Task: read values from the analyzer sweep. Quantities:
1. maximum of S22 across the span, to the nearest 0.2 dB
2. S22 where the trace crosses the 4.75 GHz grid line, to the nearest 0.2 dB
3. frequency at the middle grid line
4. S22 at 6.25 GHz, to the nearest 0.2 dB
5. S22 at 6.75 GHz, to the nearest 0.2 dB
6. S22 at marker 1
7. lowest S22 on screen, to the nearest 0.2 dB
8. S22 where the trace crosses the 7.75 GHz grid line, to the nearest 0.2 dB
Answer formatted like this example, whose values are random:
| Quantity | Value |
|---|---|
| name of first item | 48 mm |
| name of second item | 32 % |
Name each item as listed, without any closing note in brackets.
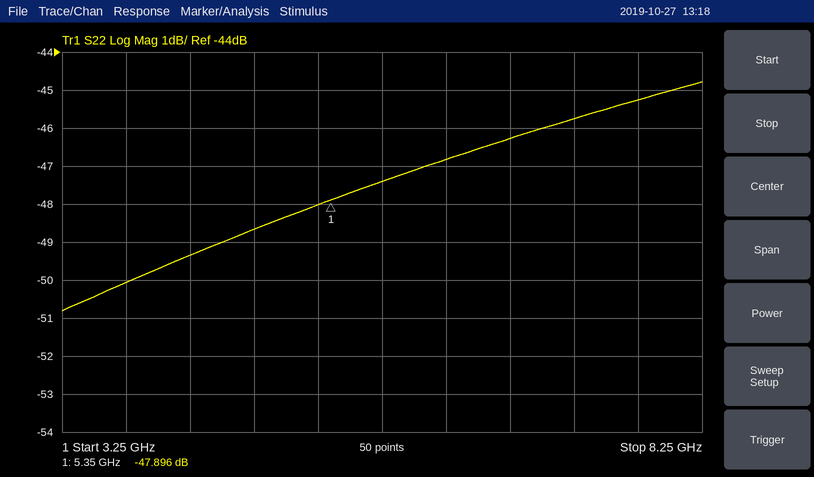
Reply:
| Quantity | Value |
|---|---|
| maximum of S22 across the span, to the nearest 0.2 dB | -44.8 dB |
| S22 where the trace crosses the 4.75 GHz grid line, to the nearest 0.2 dB | -48.6 dB |
| frequency at the middle grid line | 5.75 GHz |
| S22 at 6.25 GHz, to the nearest 0.2 dB | -46.8 dB |
| S22 at 6.75 GHz, to the nearest 0.2 dB | -46.2 dB |
| S22 at marker 1 | -47.896 dB |
| lowest S22 on screen, to the nearest 0.2 dB | -50.8 dB |
| S22 where the trace crosses the 7.75 GHz grid line, to the nearest 0.2 dB | -45.2 dB |
